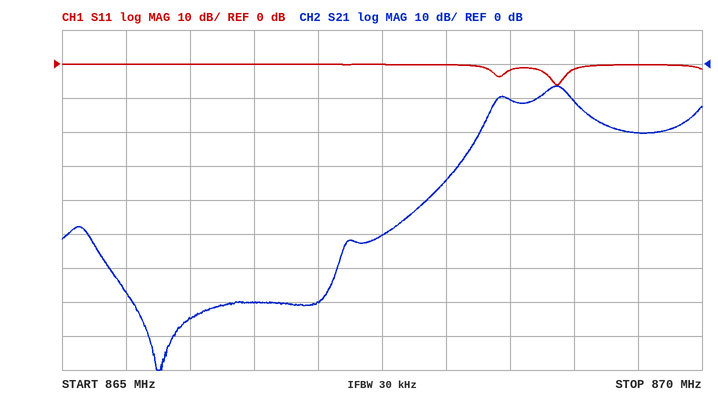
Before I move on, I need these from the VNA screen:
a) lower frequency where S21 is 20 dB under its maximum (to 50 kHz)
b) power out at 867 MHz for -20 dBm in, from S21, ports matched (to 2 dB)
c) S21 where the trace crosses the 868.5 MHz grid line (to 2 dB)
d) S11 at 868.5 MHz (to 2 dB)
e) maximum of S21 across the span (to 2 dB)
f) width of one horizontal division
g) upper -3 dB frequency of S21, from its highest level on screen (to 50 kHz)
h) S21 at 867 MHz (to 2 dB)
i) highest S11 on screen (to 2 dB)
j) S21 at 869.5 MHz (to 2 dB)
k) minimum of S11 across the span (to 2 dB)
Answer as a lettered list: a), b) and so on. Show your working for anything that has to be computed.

a) 868.15 MHz
b) -20 dBm + (-70 dB) = -90 dBm
c) -10 dB
d) -2 dB
e) -6 dB
f) 500 kHz
g) 868.95 MHz
h) -70 dB
i) 0 dB
j) -20 dB
k) -6 dB
